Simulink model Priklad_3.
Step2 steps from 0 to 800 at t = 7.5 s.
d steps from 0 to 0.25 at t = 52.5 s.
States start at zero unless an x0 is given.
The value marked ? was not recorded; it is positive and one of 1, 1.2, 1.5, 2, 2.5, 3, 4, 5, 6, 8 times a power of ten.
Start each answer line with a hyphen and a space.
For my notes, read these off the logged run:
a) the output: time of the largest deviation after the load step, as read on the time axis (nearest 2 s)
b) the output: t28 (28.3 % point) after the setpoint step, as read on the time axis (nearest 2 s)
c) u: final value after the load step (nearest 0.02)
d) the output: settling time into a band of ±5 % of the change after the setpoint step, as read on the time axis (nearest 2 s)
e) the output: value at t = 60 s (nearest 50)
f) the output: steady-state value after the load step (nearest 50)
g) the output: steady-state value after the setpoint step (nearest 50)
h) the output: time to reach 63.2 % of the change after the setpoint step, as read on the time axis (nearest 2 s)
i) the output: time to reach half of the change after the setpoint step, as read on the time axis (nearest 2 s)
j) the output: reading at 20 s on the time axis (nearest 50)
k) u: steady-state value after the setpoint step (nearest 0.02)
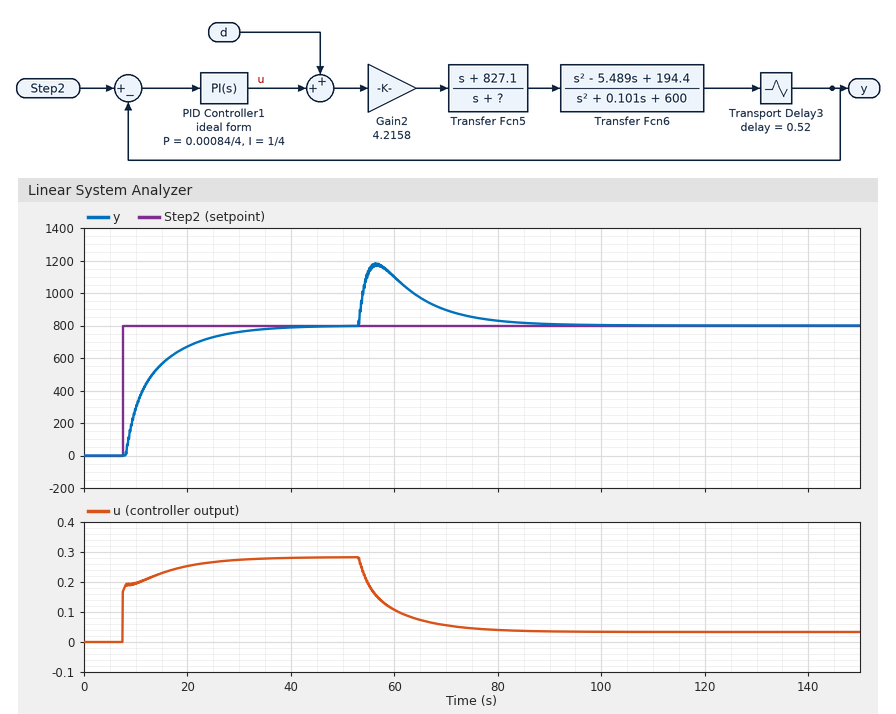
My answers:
- 56 s
- 10 s
- 0.04
- 30 s
- 1100
- 800
- 800
- 14 s
- 12 s
- 650
- 0.28
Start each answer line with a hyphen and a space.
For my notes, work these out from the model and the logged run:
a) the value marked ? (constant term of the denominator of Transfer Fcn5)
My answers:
- 0.4
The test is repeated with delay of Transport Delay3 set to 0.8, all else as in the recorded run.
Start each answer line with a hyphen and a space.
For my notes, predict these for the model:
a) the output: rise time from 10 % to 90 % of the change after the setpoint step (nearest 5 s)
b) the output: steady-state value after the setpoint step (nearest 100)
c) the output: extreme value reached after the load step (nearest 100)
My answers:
- 15 s
- 800
- 1200
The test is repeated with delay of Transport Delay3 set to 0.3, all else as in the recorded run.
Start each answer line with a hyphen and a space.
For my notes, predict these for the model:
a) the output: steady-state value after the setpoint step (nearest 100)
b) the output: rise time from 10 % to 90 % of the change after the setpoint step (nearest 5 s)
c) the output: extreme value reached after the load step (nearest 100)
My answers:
- 800
- 15 s
- 1200
